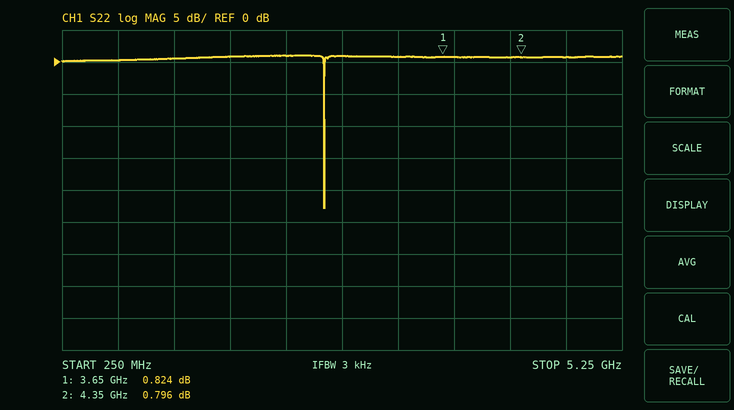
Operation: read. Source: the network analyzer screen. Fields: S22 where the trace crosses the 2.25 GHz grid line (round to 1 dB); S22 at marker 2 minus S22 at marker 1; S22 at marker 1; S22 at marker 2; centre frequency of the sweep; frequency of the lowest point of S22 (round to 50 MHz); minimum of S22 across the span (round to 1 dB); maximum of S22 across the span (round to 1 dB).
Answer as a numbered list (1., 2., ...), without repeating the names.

1. 1 dB
2. -0.028 dB
3. 0.824 dB
4. 0.796 dB
5. 2.75 GHz
6. 2.60 GHz
7. -23 dB
8. 1 dB
